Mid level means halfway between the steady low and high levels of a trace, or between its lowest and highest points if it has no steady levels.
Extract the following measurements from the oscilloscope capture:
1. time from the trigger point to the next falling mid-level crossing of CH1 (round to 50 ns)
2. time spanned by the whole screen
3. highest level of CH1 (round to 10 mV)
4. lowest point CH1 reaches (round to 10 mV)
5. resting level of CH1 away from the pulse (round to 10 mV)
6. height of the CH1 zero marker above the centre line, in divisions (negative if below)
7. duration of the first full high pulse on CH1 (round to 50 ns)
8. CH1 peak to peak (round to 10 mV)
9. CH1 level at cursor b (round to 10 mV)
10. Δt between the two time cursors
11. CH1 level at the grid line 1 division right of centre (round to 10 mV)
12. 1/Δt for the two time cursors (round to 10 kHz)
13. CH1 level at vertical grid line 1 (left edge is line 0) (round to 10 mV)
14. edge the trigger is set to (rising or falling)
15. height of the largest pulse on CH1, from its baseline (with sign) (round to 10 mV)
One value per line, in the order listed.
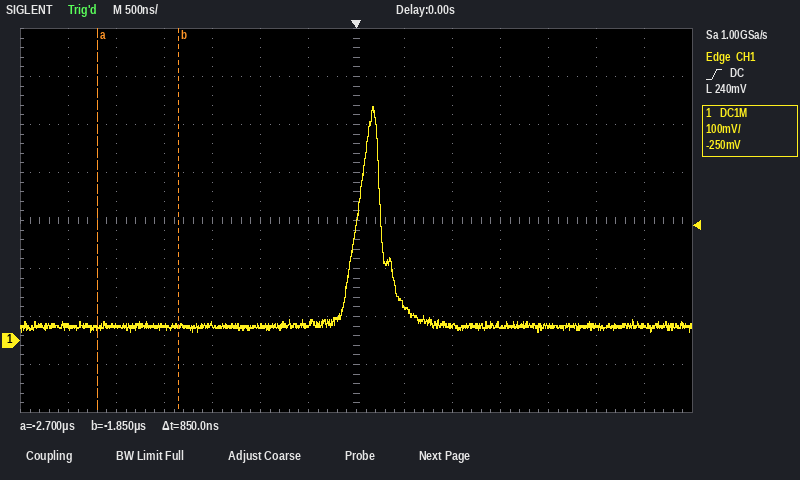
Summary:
250 ns
7 µs
490 mV
20 mV
30 mV
-2.5 div
250 ns
470 mV
30 mV
850 ns
70 mV
1.18 MHz
30 mV
rising
+460 mV
